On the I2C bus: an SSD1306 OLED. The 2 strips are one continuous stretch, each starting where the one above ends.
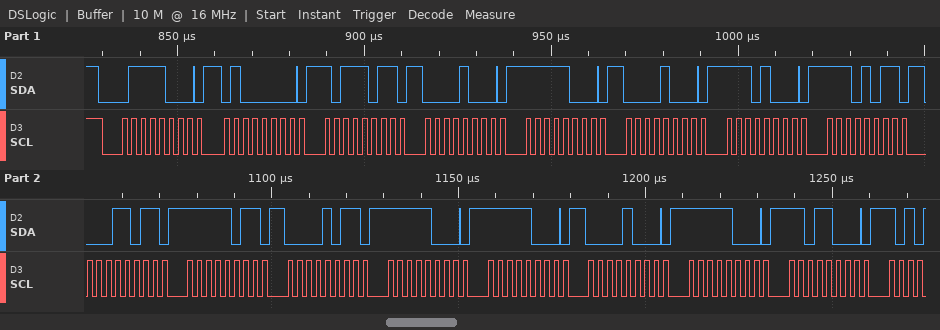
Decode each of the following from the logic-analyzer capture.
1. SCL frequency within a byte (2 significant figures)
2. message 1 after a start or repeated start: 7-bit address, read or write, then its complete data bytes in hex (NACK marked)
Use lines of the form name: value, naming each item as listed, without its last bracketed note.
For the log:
SCL frequency within a byte: 400 kHz
message 1 after a start or repeated start: 7-bit address, read or write, then its complete data bytes in hex: 0x3C write: 40 BB 08 F8 08 E8 EB 1B FB 0B F8 F8 08 F8 D8
